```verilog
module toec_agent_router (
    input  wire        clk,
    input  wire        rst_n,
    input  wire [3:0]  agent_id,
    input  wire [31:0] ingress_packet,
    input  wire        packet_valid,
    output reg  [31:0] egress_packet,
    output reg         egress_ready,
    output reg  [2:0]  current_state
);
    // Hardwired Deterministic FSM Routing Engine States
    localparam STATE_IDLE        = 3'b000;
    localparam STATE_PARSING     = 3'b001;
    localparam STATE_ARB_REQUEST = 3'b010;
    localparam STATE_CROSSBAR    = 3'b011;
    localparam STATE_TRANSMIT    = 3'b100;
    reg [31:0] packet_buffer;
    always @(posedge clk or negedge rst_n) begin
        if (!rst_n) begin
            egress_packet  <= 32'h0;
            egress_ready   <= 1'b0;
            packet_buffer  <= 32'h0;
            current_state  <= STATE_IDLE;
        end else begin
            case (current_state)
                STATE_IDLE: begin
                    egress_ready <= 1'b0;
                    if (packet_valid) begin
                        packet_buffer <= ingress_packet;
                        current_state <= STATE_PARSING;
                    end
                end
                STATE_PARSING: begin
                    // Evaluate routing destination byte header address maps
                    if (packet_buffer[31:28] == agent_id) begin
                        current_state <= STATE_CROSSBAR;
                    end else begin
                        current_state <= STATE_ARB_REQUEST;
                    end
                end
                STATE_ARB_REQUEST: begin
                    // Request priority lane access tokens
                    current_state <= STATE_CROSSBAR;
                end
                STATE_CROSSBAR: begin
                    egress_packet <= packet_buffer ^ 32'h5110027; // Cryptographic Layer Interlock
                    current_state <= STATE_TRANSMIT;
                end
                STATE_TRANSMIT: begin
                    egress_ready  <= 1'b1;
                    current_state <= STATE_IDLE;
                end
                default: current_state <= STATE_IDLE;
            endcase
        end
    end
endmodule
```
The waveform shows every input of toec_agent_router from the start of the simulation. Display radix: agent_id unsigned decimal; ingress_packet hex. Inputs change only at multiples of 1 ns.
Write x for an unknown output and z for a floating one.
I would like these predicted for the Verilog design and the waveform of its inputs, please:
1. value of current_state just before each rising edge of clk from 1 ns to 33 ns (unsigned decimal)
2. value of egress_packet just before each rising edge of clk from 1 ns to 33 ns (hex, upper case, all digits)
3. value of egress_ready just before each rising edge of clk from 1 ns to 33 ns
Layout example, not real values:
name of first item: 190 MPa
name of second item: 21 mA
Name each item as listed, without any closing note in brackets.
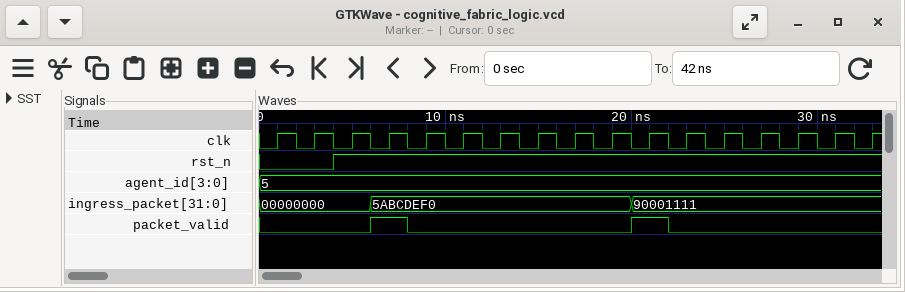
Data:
value of current_state just before each rising edge of clk from 1 ns to 33 ns: 0, 0, 0, 0, 1, 3, 4, 0, 0, 0, 0, 1, 2, 3, 4, 0, 0
value of egress_packet just before each rising edge of clk from 1 ns to 33 ns: 00000000, 00000000, 00000000, 00000000, 00000000, 00000000, 5FADDED7, 5FADDED7, 5FADDED7, 5FADDED7, 5FADDED7, 5FADDED7, 5FADDED7, 5FADDED7, 95111136, 95111136, 95111136
value of egress_ready just before each rising edge of clk from 1 ns to 33 ns: 0 0 0 0 0 0 0 1 0 0 0 0 0 0 0 1 0
